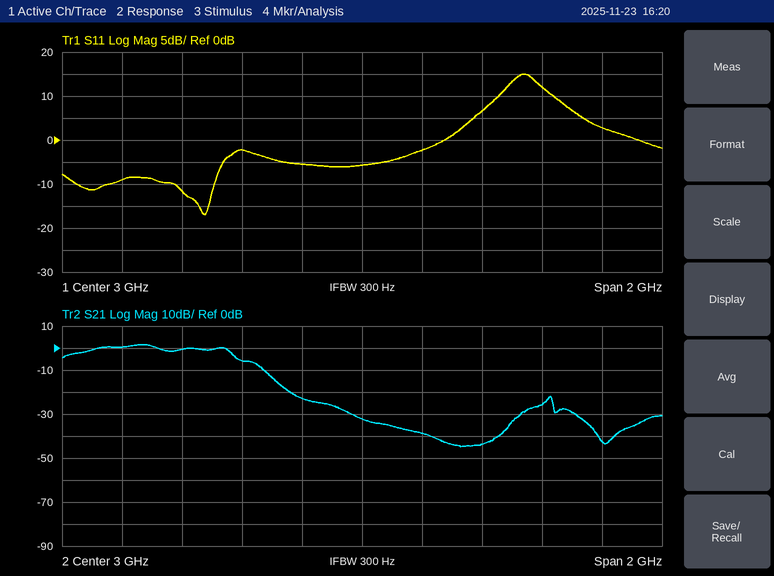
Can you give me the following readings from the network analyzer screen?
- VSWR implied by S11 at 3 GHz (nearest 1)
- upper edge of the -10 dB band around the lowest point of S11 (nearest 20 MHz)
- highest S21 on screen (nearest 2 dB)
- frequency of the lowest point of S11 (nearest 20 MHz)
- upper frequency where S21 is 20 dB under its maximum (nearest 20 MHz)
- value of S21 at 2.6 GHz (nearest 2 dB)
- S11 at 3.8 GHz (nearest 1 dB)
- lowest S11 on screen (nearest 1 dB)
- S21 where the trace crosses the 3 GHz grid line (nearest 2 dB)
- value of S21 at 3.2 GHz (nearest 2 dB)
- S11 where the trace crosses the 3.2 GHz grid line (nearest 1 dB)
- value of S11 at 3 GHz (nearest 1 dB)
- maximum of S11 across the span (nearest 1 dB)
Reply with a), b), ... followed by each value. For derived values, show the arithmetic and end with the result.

a) |Γ| = 10^(-6/20) = 0.5012; VSWR = (1 + 0.5012)/(1 − 0.5012) ≈ 3
b) 2.50 GHz
c) 2 dB
d) 2.48 GHz
e) 2.74 GHz
f) -6 dB
g) 3 dB
h) -17 dB
i) -32 dB
j) -38 dB
k) -2 dB
l) -6 dB
m) 15 dB
